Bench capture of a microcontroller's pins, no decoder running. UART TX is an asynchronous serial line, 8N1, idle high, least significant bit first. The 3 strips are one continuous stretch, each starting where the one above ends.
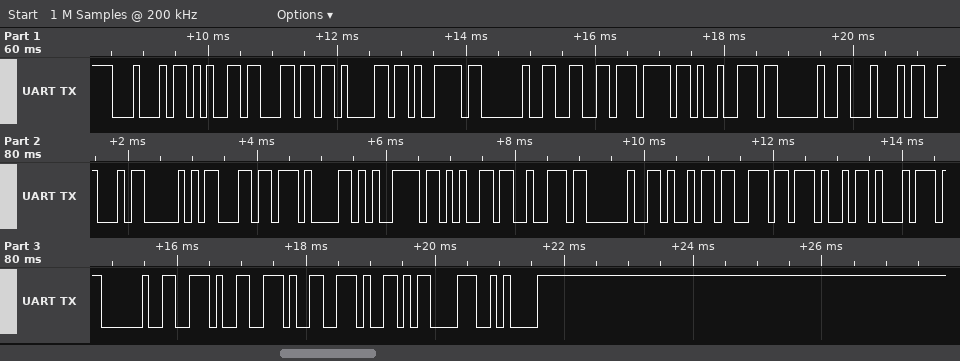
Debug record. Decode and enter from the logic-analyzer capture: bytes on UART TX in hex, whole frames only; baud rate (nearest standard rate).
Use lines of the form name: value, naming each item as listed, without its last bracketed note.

bytes on UART TX in hex, whole frames only: 44 65 6C 61 79 20 66 6F 72 20 44 46 50 6C 61 79 65 72 20 69 6E 69 74 20 2E 2E 2E 0D 0A
baud rate: 9600 baud
